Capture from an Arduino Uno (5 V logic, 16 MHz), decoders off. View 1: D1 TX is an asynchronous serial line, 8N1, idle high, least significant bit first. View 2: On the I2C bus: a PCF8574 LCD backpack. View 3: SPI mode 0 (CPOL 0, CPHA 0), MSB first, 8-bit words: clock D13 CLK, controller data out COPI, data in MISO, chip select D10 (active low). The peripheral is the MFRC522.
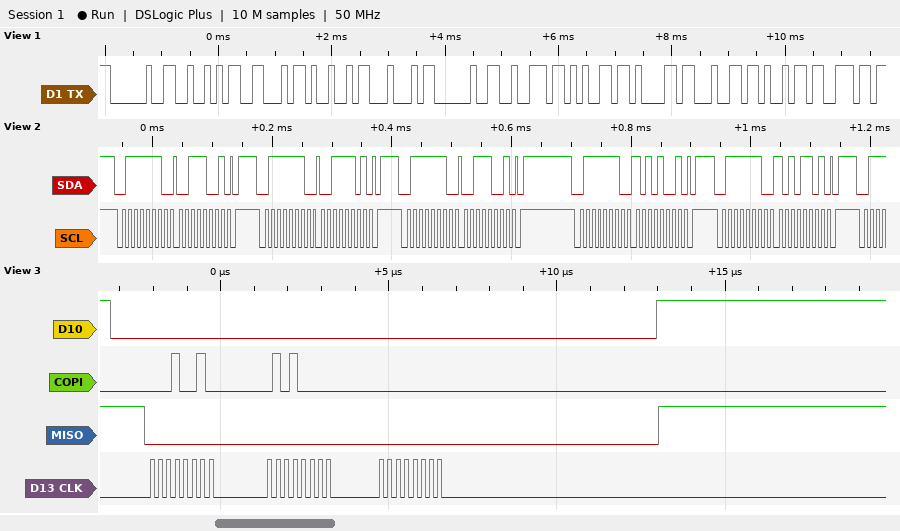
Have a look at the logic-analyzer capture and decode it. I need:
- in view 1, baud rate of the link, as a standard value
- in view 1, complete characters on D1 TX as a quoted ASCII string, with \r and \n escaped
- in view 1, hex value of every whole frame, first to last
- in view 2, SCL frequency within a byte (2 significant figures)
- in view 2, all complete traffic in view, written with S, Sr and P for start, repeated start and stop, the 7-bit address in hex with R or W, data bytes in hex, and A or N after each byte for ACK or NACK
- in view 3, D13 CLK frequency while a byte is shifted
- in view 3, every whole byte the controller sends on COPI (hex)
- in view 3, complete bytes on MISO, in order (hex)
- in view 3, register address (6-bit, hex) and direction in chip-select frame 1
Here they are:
9600 baud
" RFID readin"
0x20 0x52 0x46 0x49 0x44 0x20 0x72 0x65 0x61 0x64 0x69 0x6E
100 kHz
S 3FW A 39 A P S 3FW A 3D A P S 3FW A 39 A P S 3FW A A9 A P S 3FW A AD A P
4 MHz
0x12 0x50 0x00
0x00 0x00 0x00
0x09 write
